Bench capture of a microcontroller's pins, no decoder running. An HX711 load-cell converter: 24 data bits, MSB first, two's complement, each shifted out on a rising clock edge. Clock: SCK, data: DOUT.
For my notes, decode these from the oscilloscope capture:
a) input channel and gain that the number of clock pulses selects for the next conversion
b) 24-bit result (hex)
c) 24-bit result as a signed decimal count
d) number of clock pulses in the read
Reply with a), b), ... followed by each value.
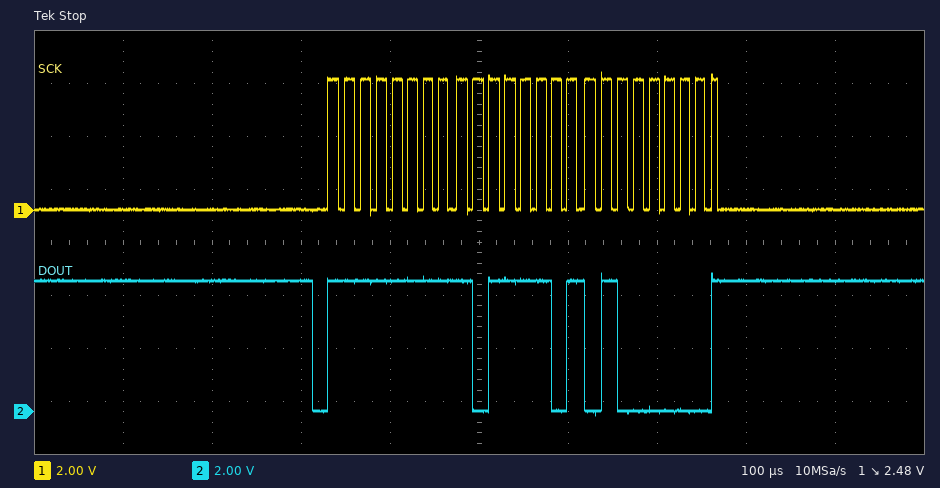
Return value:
a) channel A, gain 128
b) 0xFFBD40
c) -17088
d) 25
